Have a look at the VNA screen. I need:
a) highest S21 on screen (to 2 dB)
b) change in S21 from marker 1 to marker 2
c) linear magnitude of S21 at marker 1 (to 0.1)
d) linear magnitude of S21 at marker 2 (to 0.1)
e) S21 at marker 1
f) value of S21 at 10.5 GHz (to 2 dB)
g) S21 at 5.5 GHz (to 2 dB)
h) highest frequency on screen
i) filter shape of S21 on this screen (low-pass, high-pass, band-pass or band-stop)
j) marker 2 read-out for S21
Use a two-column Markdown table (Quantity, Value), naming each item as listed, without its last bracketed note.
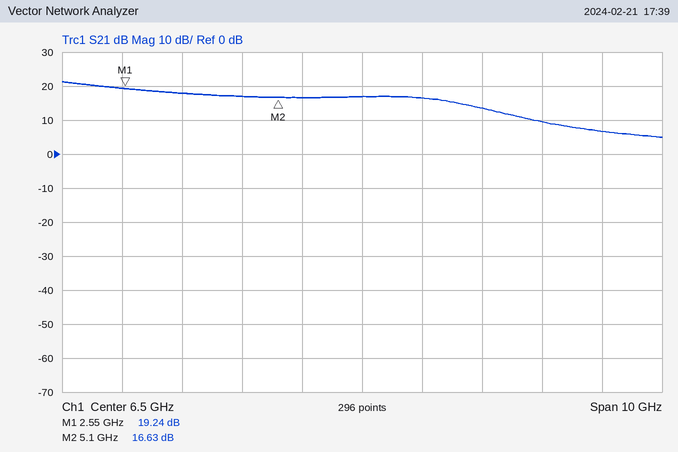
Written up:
| Quantity | Value |
|---|---|
| highest S21 on screen | 22 dB |
| change in S21 from marker 1 to marker 2 | -2.61 dB |
| linear magnitude of S21 at marker 1 | 9.2 |
| linear magnitude of S21 at marker 2 | 6.8 |
| S21 at marker 1 | 19.24 dB |
| value of S21 at 10.5 GHz | 6 dB |
| S21 at 5.5 GHz | 16 dB |
| highest frequency on screen | 11.5 GHz |
| filter shape of S21 on this screen | low-pass |
| marker 2 read-out for S21 | 16.63 dB |
